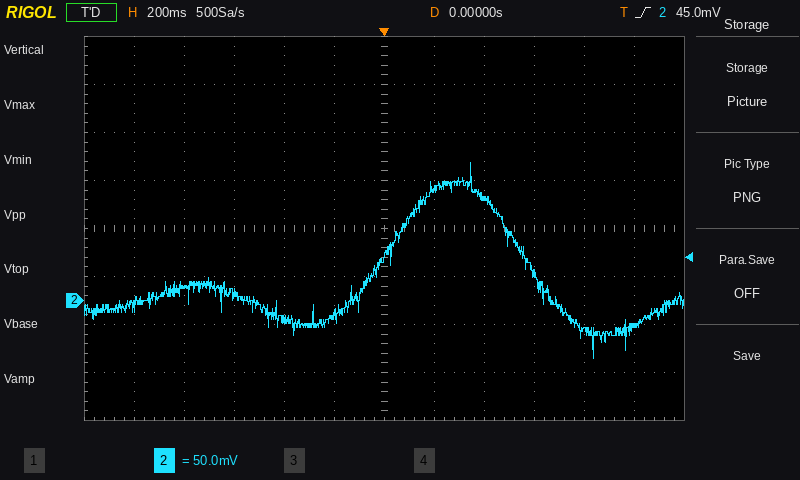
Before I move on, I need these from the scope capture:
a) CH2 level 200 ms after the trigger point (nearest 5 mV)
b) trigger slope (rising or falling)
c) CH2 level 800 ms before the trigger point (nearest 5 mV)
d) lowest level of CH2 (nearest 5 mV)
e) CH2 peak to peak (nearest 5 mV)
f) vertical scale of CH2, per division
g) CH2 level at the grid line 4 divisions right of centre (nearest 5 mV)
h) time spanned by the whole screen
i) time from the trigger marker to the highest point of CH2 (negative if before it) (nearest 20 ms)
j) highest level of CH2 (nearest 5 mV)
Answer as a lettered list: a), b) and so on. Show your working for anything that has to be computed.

a) 115 mV
b) rising
c) 15 mV
d) -60 mV
e) 145 mV − (-60 mV) = 205 mV
f) 50 mV
g) -30 mV
h) 2.4 s
i) +340 ms
j) 145 mV
